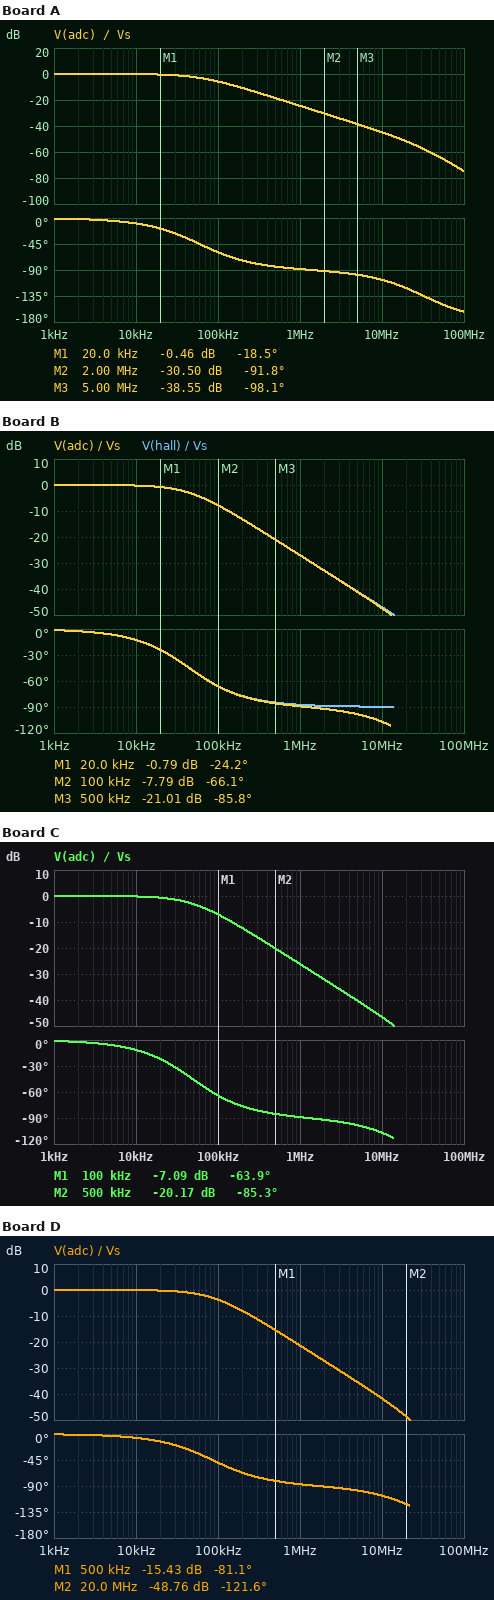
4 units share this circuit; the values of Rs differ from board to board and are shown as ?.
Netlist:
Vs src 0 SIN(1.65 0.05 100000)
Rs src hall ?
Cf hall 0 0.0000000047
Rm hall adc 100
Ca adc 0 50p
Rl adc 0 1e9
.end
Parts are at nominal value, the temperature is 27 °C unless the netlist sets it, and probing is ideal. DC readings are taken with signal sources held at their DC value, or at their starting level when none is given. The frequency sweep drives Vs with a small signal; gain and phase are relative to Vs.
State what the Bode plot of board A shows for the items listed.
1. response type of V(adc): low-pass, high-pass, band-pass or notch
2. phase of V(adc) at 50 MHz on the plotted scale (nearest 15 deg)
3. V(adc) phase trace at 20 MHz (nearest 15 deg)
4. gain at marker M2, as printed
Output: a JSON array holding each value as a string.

["low-pass", "-150 deg", "-120 deg", "-30.50 dB"]
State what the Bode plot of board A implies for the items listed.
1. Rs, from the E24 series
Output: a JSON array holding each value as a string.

["560 Ω"]
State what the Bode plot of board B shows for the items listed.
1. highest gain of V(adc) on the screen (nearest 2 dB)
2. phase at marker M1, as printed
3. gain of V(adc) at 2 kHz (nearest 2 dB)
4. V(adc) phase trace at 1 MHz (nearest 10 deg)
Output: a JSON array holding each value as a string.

["0 dB", "-24.2 deg", "0 dB", "-90 deg"]
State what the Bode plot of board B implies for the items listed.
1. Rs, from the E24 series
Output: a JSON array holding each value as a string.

["750 Ω"]
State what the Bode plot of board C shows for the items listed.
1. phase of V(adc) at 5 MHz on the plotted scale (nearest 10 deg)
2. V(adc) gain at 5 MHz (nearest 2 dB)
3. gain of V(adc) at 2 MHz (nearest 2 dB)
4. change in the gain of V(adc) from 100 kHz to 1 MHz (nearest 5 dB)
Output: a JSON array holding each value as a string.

["-100 deg", "-40 dB", "-32 dB", "-20 dB"]
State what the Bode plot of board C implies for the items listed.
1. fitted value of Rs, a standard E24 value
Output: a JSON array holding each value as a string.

["680 Ω"]
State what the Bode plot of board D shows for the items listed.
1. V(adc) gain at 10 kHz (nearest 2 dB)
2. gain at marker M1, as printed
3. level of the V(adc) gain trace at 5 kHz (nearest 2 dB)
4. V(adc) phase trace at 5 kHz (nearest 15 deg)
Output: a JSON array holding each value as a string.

["0 dB", "-15.43 dB", "0 dB", "0 deg"]
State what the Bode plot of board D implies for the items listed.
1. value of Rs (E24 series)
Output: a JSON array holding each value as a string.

["390 Ω"]
